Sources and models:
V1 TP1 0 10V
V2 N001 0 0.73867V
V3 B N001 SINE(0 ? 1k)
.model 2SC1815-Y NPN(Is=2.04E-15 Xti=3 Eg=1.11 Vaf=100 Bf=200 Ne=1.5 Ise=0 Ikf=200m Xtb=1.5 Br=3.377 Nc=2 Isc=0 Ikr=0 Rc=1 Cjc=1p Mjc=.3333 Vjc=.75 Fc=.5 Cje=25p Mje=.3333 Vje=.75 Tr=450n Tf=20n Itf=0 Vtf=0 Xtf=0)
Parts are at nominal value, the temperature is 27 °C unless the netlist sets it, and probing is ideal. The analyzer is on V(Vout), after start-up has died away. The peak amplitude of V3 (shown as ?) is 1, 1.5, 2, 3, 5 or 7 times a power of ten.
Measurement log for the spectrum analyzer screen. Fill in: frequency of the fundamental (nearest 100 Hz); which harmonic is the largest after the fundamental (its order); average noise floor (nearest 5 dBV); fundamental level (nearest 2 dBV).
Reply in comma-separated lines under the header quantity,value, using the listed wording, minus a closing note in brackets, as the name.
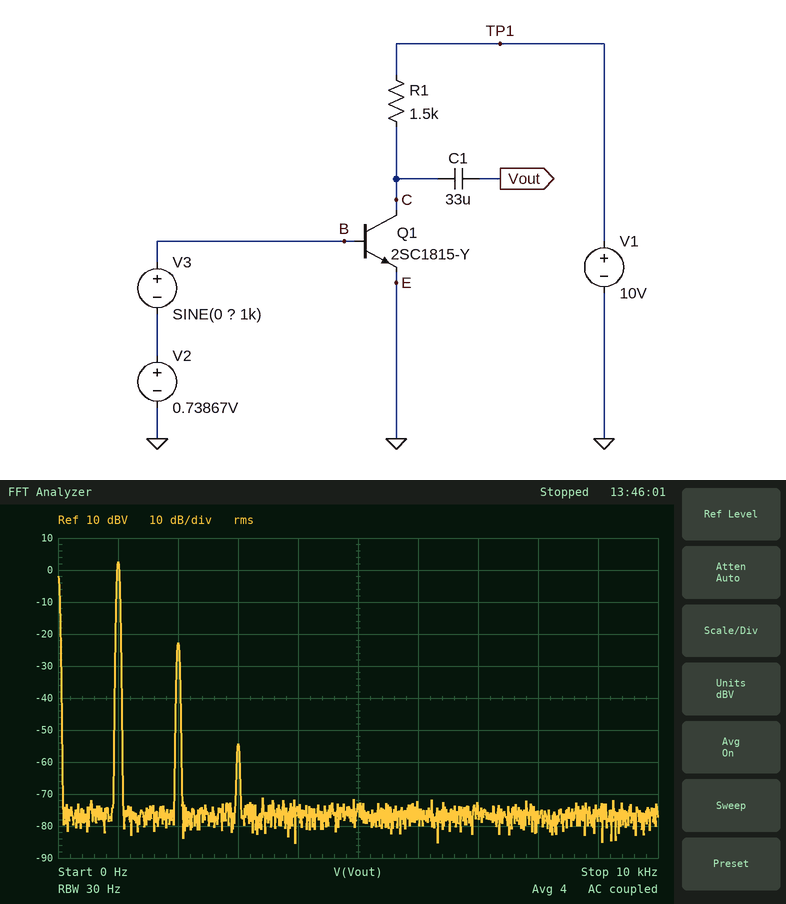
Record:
quantity,value
frequency of the fundamental,1.0 kHz
which harmonic is the largest after the fundamental,2
average noise floor,-75 dBV
fundamental level,2 dBV
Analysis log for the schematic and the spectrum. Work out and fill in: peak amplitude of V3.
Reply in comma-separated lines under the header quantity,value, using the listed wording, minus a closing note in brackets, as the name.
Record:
quantity,value
peak amplitude of V3,7 mV
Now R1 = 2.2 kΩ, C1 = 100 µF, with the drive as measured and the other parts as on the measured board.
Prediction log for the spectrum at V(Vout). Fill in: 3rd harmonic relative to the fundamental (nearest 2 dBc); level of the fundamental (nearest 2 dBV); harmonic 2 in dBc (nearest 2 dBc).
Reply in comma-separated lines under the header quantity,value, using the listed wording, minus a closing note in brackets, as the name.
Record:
quantity,value
3rd harmonic relative to the fundamental,-14 dBc
level of the fundamental,-8 dBV
harmonic 2 in dBc,-4 dBc
